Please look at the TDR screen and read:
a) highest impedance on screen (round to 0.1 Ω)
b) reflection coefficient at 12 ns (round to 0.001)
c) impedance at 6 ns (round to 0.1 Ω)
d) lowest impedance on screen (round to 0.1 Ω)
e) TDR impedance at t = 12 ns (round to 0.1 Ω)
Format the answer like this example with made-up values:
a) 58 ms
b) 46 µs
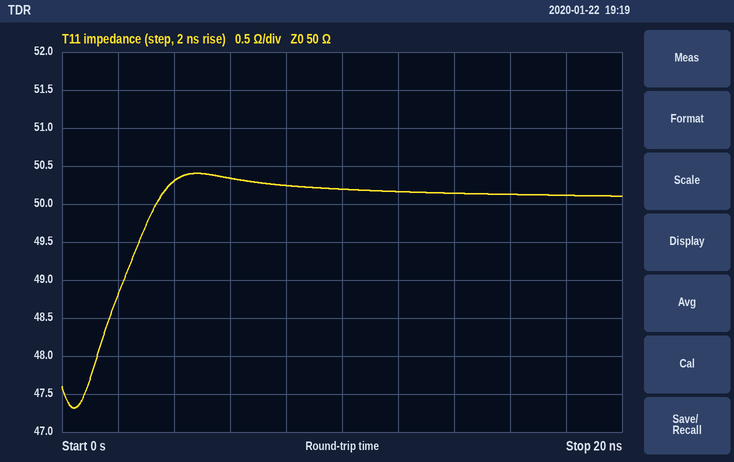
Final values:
a) 50.4 Ω
b) +0.002
c) 50.3 Ω
d) 47.3 Ω
e) 50.2 Ω
